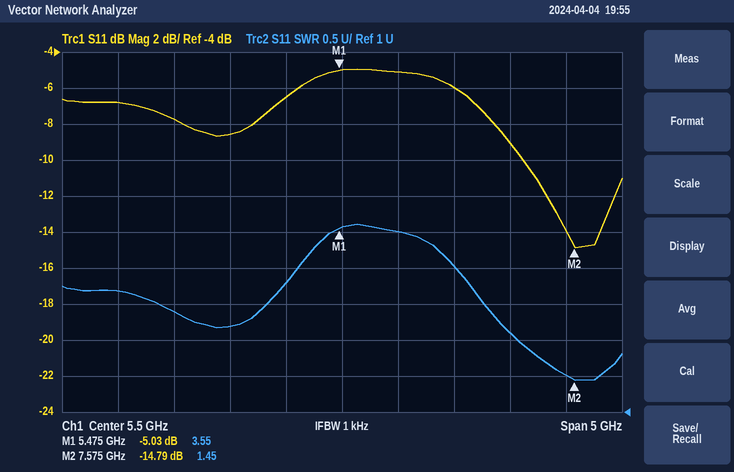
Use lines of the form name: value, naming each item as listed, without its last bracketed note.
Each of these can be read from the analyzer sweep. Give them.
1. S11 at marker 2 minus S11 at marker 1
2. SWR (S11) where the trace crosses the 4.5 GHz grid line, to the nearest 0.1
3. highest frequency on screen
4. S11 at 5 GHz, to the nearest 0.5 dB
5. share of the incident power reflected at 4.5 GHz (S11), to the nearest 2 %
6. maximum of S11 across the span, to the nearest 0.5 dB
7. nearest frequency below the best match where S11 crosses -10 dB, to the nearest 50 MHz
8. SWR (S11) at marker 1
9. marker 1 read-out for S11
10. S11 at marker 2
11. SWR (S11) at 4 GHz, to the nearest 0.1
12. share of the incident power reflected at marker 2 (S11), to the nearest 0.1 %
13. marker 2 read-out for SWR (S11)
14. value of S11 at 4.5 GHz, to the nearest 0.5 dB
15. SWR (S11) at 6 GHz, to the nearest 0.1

S11 at marker 2 minus S11 at marker 1: -9.76 dB
SWR (S11) where the trace crosses the 4.5 GHz grid line, to the nearest 0.1: 2.2
highest frequency on screen: 8 GHz
S11 at 5 GHz, to the nearest 0.5 dB: -6.5 dB
share of the incident power reflected at 4.5 GHz (S11), to the nearest 2 %: 14 %
maximum of S11 across the span, to the nearest 0.5 dB: -5.0 dB
nearest frequency below the best match where S11 crosses -10 dB, to the nearest 50 MHz: 7.10 GHz
SWR (S11) at marker 1: 3.55
marker 1 read-out for S11: -5.03 dB
S11 at marker 2: -14.79 dB
SWR (S11) at 4 GHz, to the nearest 0.1: 2.4
share of the incident power reflected at marker 2 (S11), to the nearest 0.1 %: 3.3 %
marker 2 read-out for SWR: 1.45
value of S11 at 4.5 GHz, to the nearest 0.5 dB: -8.5 dB
SWR (S11) at 6 GHz, to the nearest 0.1: 3.5
